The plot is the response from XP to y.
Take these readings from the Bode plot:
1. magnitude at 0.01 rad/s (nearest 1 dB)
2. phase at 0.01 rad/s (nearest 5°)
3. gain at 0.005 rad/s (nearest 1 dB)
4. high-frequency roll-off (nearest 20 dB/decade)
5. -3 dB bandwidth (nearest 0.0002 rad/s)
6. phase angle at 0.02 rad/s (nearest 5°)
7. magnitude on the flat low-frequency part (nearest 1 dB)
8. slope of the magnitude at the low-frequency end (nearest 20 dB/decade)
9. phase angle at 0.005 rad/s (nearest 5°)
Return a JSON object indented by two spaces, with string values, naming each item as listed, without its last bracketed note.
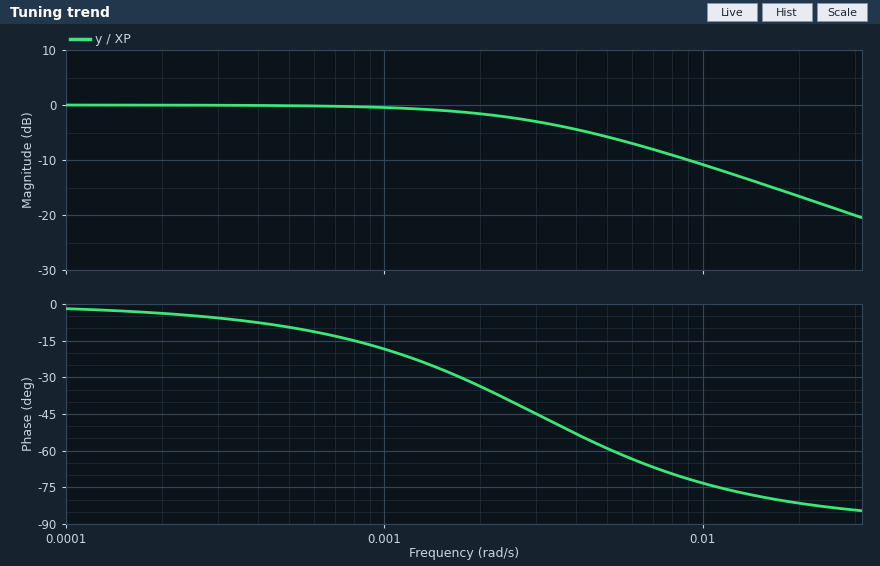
{
  "magnitude at 0.01 rad/s": "-11 dB",
  "phase at 0.01 rad/s": "-75°",
  "gain at 0.005 rad/s": "-6 dB",
  "high-frequency roll-off": "-20 dB/decade",
  "-3 dB bandwidth": "0.0030 rad/s",
  "phase angle at 0.02 rad/s": "-80°",
  "magnitude on the flat low-frequency part": "0 dB",
  "slope of the magnitude at the low-frequency end": "0 dB/decade",
  "phase angle at 0.005 rad/s": "-60°"
}
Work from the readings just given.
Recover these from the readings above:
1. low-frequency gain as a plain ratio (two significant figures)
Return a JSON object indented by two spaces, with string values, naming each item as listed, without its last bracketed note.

{
  "low-frequency gain as a plain ratio": "1.0"
}
